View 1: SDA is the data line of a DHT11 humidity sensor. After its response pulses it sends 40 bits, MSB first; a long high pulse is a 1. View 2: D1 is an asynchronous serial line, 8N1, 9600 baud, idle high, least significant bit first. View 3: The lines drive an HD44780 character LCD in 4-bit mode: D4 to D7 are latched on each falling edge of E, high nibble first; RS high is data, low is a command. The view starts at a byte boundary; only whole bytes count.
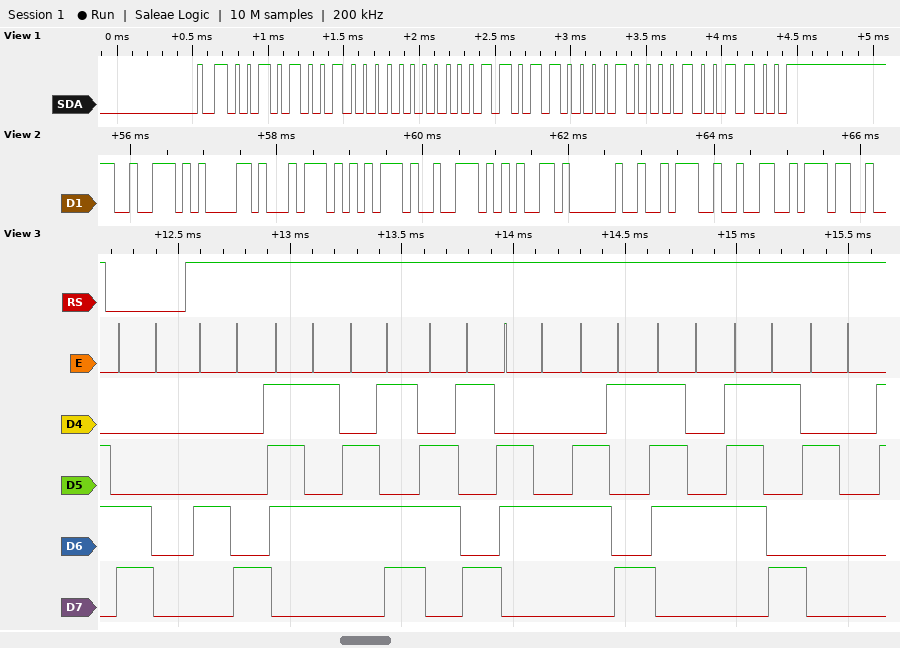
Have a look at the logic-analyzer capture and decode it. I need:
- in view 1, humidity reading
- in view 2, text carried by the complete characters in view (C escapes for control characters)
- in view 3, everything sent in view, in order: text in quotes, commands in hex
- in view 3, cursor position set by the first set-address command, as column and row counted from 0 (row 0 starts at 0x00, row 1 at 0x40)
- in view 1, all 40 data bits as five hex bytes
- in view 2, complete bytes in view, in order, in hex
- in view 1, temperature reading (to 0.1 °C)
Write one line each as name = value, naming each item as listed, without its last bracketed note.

in view 1, humidity reading = 41 %
in view 2, text carried by the complete characters in view = "rature :27"
in view 3, everything sent in view, in order: text in quotes, commands in hex = 0xC0 "Humidity "
in view 3, cursor position set by the first set-address command, as column and row counted from 0 = column 0, row 1
in view 1, all 40 data bits as five hex bytes = 29 00 1B 08 4C
in view 2, complete bytes in view, in order, in hex = 72 61 74 75 72 65 20 3A 32 37
in view 1, temperature reading = 27.8 °C
